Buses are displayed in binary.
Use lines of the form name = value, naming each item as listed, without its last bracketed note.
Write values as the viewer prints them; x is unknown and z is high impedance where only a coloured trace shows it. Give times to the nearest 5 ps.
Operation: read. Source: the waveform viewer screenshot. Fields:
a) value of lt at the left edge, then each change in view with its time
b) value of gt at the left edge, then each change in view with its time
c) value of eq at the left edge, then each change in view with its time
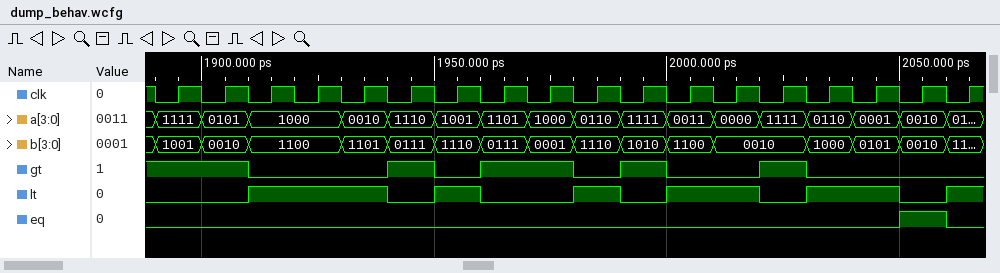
value of lt at the left edge, then each change in view with its time = 0, 1 at 1910 ps, 0 at 1940 ps, 1 at 1950 ps, 0 at 1960 ps, 1 at 1980 ps, 0 at 1990 ps, 1 at 2000 ps, 0 at 2020 ps, 1 at 2030 ps, 0 at 2050 ps, 1 at 2060 ps
value of gt at the left edge, then each change in view with its time = 1, 0 at 1910 ps, 1 at 1940 ps, 0 at 1950 ps, 1 at 1960 ps, 0 at 1980 ps, 1 at 1990 ps, 0 at 2000 ps, 1 at 2020 ps, 0 at 2030 ps
value of eq at the left edge, then each change in view with its time = 0, 1 at 2050 ps, 0 at 2060 ps
